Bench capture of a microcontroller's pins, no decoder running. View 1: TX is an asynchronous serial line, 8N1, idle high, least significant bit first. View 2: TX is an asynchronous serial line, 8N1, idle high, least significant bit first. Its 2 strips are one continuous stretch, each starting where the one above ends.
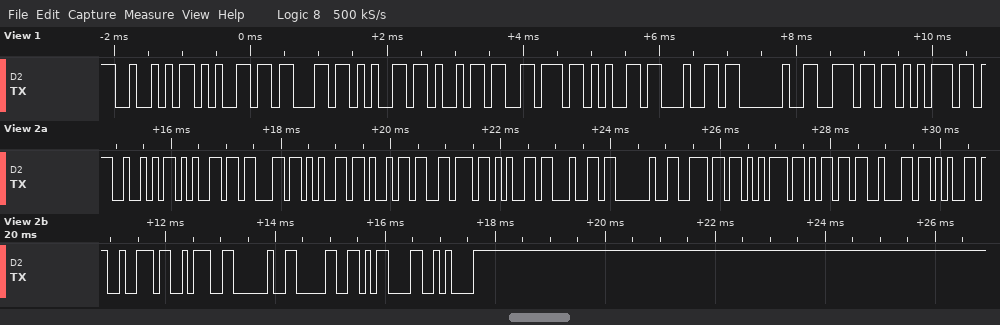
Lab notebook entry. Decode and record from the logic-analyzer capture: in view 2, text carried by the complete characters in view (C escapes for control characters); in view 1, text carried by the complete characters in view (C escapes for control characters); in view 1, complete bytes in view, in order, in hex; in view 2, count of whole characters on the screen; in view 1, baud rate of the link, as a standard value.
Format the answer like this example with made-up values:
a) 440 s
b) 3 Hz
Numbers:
a) "Received number: 0\r\n"
b) "Received nu"
c) 52 65 63 65 69 76 65 64 20 6E 75
d) 20
e) 9600 baud
